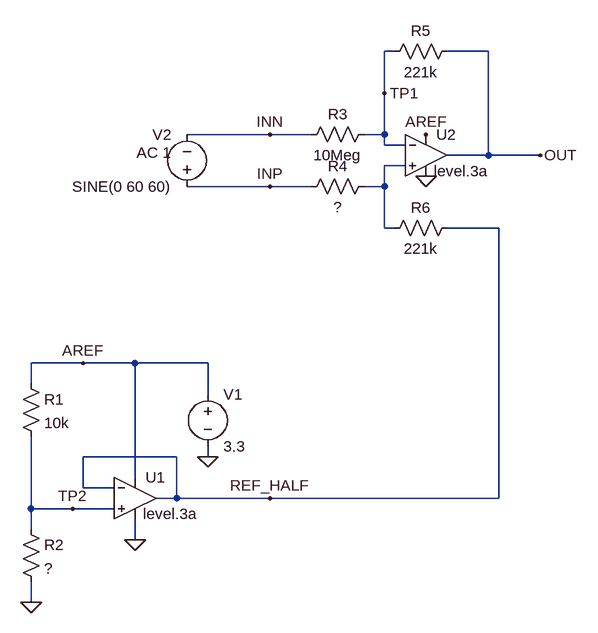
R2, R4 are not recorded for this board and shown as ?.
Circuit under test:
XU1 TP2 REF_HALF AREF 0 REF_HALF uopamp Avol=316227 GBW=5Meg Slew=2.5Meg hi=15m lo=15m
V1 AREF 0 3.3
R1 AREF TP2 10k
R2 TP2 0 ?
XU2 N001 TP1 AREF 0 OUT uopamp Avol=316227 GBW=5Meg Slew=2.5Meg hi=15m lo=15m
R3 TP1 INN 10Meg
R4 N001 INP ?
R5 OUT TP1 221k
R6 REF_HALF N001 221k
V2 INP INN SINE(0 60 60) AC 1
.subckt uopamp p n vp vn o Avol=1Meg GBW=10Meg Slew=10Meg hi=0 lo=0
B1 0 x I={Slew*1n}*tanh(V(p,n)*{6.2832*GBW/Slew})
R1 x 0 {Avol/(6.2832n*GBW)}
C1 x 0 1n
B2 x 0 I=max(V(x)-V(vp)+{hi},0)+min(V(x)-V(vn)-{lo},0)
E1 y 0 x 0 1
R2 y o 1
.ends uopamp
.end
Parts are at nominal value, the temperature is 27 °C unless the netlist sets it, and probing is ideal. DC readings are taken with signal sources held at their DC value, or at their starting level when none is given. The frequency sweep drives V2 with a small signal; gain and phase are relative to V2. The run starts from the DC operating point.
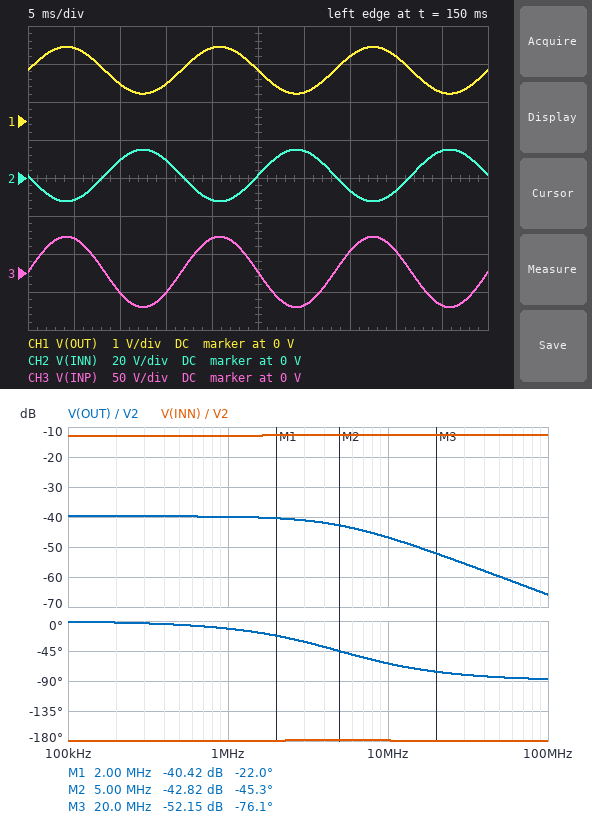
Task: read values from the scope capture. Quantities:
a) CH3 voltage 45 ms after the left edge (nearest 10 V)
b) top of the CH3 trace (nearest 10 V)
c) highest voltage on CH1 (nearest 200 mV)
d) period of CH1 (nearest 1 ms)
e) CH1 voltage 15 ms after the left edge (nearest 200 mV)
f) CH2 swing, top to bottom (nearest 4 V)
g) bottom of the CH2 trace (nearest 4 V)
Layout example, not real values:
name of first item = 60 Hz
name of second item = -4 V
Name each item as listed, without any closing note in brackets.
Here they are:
CH3 voltage 45 ms after the left edge = -40 V
top of the CH3 trace = 50 V
highest voltage on CH1 = 2.0 V
period of CH1 = 17 ms
CH1 voltage 15 ms after the left edge = 1.0 V
CH2 swing, top to bottom = 28 V
bottom of the CH2 trace = -12 V
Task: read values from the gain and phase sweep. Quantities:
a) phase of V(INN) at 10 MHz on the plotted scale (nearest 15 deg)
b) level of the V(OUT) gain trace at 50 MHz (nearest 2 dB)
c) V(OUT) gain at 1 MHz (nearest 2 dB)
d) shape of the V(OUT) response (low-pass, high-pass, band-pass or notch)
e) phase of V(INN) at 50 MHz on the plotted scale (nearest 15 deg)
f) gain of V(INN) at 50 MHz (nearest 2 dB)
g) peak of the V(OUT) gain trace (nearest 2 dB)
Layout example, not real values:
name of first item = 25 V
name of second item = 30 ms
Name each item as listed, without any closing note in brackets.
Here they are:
phase of V(INN) at 10 MHz on the plotted scale = -180 deg
level of the V(OUT) gain trace at 50 MHz = -60 dB
V(OUT) gain at 1 MHz = -40 dB
shape of the V(OUT) response = low-pass
phase of V(INN) at 50 MHz on the plotted scale = -180 deg
gain of V(INN) at 50 MHz = -12 dB
peak of the V(OUT) gain trace = -40 dB
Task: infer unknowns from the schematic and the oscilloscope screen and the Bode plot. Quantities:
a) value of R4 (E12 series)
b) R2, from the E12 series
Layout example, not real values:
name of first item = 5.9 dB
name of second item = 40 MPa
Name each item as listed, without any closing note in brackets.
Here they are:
value of R4 = 33 MΩ
R2, from the E12 series = 6.8 kΩ
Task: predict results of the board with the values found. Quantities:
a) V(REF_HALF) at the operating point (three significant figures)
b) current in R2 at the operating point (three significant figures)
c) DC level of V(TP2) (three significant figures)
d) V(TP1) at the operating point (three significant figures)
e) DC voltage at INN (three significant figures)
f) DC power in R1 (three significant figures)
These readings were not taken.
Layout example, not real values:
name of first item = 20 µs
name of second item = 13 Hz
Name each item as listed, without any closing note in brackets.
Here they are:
V(REF_HALF) at the operating point = 1.34 V
current in R2 at the operating point = 196 µA
DC level of V(TP2) = 1.34 V
V(TP1) at the operating point = 1.34 V
DC voltage at INN = 1.34 V
DC power in R1 = 386 µW
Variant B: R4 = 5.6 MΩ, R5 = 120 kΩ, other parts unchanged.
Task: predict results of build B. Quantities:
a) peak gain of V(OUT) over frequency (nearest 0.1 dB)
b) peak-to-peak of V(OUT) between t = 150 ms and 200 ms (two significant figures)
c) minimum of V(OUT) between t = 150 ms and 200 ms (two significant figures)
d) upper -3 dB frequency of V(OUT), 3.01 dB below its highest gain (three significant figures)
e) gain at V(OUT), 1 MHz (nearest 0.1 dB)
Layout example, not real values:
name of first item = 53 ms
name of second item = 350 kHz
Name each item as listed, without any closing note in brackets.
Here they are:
peak gain of V(OUT) over frequency = -33.2 dB
peak-to-peak of V(OUT) between t = 150 ms and 200 ms = 2.6 V
minimum of V(OUT) between t = 150 ms and 200 ms = 24 mV
upper -3 dB frequency of V(OUT), 3.01 dB below its highest gain = 4.89 MHz
gain at V(OUT), 1 MHz = -33.4 dB
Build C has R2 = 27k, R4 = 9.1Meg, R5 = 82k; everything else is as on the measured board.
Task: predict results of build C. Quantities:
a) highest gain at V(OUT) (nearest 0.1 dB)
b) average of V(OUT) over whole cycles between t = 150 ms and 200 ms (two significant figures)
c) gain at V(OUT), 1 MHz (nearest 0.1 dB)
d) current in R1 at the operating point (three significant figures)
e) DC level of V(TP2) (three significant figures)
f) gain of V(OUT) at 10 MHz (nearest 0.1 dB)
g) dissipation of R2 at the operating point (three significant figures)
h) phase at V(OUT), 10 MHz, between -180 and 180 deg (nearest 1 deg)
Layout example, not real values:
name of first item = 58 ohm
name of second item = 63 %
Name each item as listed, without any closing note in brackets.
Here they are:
highest gain at V(OUT) = -36.0 dB
average of V(OUT) over whole cycles between t = 150 ms and 200 ms = 2.4 V
gain at V(OUT), 1 MHz = -36.2 dB
current in R1 at the operating point = 89.2 µA
DC level of V(TP2) = 2.41 V
gain of V(OUT) at 10 MHz = -43.1 dB
dissipation of R2 at the operating point = 215 µW
phase at V(OUT), 10 MHz, between -180 and 180 deg = -64 deg
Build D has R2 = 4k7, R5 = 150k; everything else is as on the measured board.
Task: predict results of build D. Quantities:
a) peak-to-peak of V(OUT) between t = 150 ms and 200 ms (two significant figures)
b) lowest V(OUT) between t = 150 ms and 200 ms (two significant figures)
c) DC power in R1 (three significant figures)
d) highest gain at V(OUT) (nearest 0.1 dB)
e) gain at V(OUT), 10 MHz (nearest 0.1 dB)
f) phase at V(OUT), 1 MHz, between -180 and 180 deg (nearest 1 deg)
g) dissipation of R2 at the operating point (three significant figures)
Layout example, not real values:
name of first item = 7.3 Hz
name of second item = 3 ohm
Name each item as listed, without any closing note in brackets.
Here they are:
peak-to-peak of V(OUT) between t = 150 ms and 200 ms = 1.0 V
lowest V(OUT) between t = 150 ms and 200 ms = 540 mV
DC power in R1 = 504 µW
highest gain at V(OUT) = -41.3 dB
gain at V(OUT), 10 MHz = -48.3 dB
phase at V(OUT), 1 MHz, between -180 and 180 deg = -11 deg
dissipation of R2 at the operating point = 237 µW
